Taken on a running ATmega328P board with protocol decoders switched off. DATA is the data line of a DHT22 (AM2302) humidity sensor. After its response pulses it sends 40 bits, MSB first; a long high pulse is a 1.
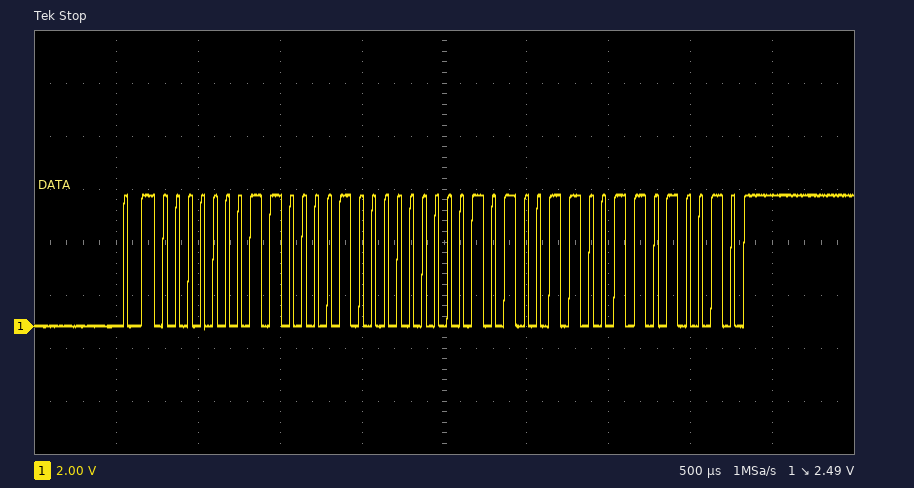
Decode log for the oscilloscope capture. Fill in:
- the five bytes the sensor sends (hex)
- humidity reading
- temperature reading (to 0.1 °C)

01 84 01 4C D2
38.8 %
33.2 °C
